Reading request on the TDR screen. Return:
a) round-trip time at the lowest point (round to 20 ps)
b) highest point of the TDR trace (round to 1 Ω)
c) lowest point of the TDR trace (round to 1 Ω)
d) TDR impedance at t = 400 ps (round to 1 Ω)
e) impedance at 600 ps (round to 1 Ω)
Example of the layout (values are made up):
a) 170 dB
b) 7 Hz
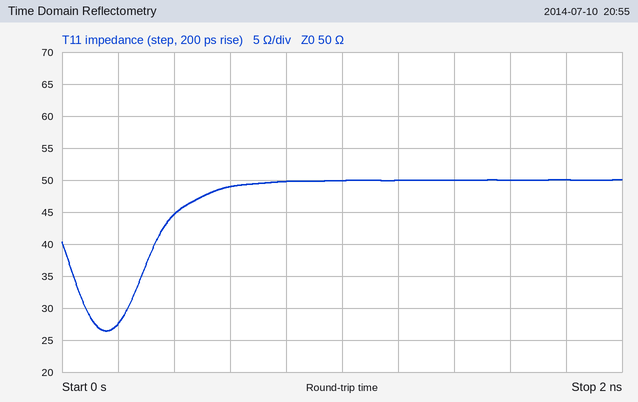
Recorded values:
a) 160 ps
b) 50 Ω
c) 26 Ω
d) 45 Ω
e) 49 Ω
